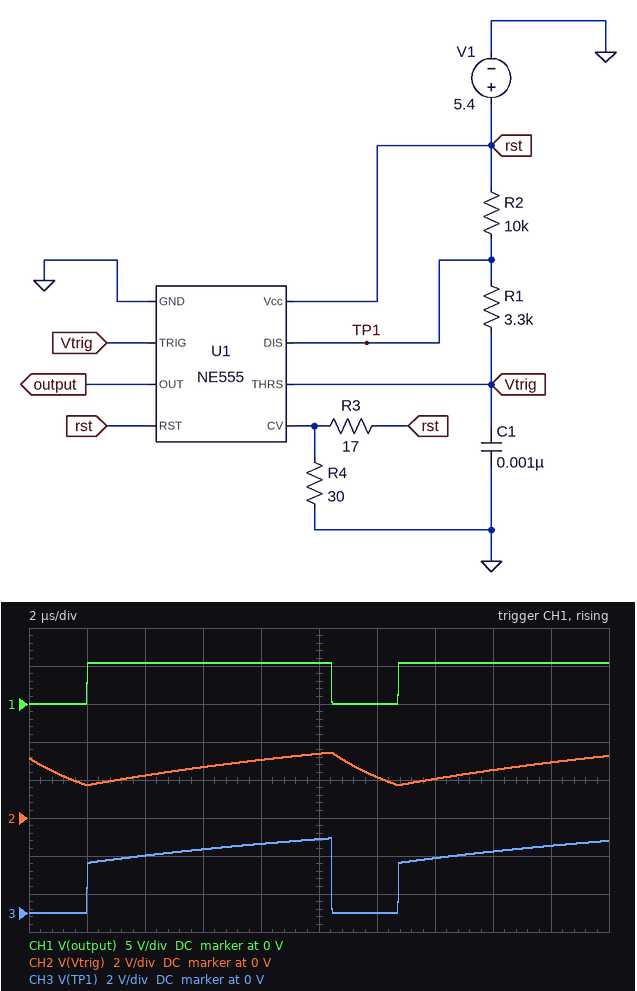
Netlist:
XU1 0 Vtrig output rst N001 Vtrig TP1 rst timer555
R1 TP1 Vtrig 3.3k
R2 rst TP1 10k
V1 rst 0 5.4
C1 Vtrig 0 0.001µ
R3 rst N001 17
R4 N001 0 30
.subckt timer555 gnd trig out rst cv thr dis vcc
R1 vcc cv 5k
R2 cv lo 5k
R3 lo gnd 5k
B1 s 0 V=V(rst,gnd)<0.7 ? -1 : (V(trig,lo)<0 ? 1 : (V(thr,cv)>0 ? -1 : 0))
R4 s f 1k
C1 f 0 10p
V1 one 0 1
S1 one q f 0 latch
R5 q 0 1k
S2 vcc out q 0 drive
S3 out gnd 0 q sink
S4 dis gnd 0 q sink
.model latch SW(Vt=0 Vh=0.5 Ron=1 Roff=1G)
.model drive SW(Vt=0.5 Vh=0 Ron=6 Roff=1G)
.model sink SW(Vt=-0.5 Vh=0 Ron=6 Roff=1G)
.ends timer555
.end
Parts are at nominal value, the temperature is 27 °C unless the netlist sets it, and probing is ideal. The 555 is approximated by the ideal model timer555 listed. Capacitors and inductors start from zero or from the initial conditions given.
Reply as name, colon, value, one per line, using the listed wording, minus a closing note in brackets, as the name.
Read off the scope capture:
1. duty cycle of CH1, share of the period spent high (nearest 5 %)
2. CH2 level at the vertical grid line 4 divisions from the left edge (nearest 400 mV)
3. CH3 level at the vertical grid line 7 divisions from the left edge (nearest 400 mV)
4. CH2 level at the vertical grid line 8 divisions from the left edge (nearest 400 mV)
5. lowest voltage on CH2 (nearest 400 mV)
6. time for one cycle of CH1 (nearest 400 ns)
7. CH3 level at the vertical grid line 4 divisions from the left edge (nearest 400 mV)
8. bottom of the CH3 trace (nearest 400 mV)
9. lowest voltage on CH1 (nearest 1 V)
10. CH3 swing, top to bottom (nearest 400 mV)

duty cycle of CH1, share of the period spent high: 80 %
CH2 level at the vertical grid line 4 divisions from the left edge: 3.2 V
CH3 level at the vertical grid line 7 divisions from the left edge: 2.8 V
CH2 level at the vertical grid line 8 divisions from the left edge: 2.4 V
lowest voltage on CH2: 1.6 V
time for one cycle of CH1: 10.8 µs
CH3 level at the vertical grid line 4 divisions from the left edge: 3.6 V
bottom of the CH3 trace: 0 V
lowest voltage on CH1: 0 V
CH3 swing, top to bottom: 4.0 V
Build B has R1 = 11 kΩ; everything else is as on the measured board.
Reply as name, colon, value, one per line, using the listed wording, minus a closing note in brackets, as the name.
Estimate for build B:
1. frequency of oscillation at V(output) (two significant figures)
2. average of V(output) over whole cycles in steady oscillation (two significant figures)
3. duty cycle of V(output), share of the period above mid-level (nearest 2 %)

frequency of oscillation at V(output): 48 kHz
average of V(output) over whole cycles in steady oscillation: 3.4 V
duty cycle of V(output), share of the period above mid-level: 64 %
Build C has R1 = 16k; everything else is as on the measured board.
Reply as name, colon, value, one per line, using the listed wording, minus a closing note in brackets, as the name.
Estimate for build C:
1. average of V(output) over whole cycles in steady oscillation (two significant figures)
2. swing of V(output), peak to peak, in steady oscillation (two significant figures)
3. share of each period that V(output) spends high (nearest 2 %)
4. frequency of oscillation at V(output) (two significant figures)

average of V(output) over whole cycles in steady oscillation: 3.2 V
swing of V(output), peak to peak, in steady oscillation: 5.4 V
share of each period that V(output) spends high: 60 %
frequency of oscillation at V(output): 36 kHz
